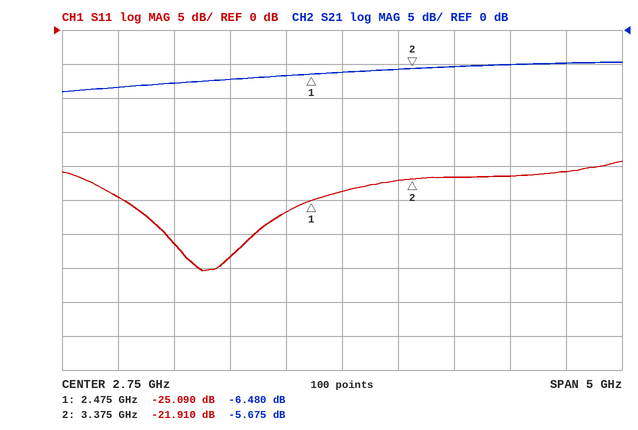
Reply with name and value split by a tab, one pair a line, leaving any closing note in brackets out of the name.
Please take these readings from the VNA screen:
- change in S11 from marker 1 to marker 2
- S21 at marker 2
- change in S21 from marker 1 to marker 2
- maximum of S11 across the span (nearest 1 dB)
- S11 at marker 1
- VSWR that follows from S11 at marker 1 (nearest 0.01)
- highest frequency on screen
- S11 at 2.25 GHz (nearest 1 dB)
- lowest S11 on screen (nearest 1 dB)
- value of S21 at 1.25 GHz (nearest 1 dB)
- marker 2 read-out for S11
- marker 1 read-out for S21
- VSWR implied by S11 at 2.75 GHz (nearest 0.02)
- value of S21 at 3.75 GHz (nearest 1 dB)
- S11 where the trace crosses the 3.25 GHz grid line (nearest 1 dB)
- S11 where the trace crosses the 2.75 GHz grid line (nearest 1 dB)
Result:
change in S11 from marker 1 to marker 2	3.180 dB
S21 at marker 2	-5.675 dB
change in S21 from marker 1 to marker 2	0.805 dB
maximum of S11 across the span	-19 dB
S11 at marker 1	-25.090 dB
VSWR that follows from S11 at marker 1	1.12
highest frequency on screen	5.25 GHz
S11 at 2.25 GHz	-27 dB
lowest S11 on screen	-35 dB
value of S21 at 1.25 GHz	-8 dB
marker 2 read-out for S11	-21.910 dB
marker 1 read-out for S21	-6.480 dB
VSWR implied by S11 at 2.75 GHz	1.14
value of S21 at 3.75 GHz	-5 dB
S11 where the trace crosses the 3.25 GHz grid line	-22 dB
S11 where the trace crosses the 2.75 GHz grid line	-24 dB
